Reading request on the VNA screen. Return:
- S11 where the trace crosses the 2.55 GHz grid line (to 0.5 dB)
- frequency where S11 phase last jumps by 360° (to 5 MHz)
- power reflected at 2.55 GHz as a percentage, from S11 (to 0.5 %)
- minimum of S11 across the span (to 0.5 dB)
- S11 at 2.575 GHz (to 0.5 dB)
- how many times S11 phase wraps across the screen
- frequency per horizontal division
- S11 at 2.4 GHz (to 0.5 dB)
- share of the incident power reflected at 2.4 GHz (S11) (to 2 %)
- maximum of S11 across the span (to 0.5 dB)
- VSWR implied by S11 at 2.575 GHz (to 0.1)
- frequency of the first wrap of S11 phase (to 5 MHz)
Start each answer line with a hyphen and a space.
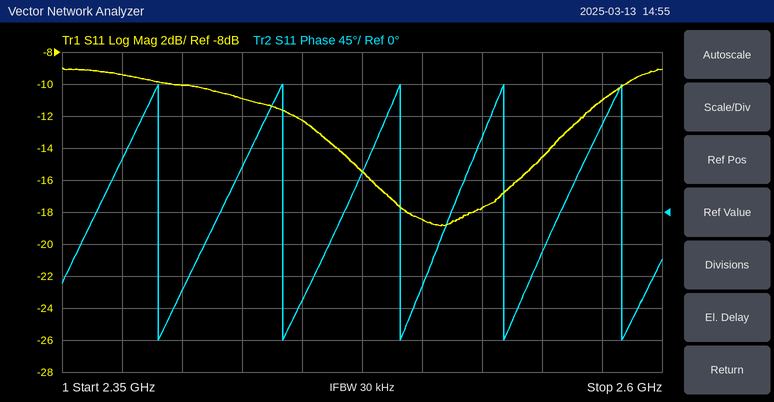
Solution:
- -14.5 dB
- 2.585 GHz
- 3.5 %
- -19.0 dB
- -11.0 dB
- 5
- 25 MHz
- -10.0 dB
- 10 %
- -9.0 dB
- 1.8
- 2.390 GHz
